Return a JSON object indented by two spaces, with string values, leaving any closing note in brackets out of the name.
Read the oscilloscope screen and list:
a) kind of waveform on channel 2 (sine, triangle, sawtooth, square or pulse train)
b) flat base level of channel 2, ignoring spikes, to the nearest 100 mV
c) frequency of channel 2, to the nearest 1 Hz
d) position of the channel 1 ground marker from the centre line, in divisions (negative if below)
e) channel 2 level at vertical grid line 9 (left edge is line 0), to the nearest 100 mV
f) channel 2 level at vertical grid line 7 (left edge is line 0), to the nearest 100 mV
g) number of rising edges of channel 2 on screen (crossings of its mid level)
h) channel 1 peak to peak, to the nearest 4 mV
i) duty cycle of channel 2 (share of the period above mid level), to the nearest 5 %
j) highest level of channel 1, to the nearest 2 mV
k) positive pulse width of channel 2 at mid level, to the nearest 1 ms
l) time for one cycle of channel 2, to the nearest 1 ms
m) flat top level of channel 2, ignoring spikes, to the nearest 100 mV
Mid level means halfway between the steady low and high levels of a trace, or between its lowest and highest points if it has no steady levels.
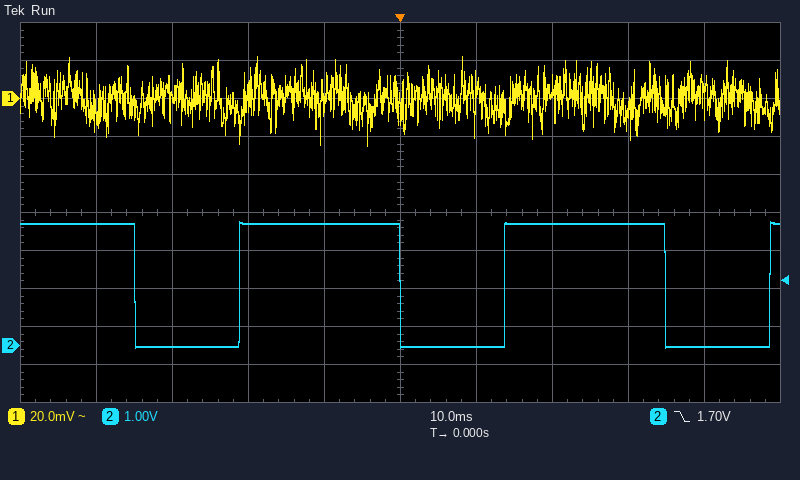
{
  "kind of waveform on channel 2": "pulse train",
  "flat base level of channel 2, ignoring spikes, to the nearest 100 mV": "0.0 V",
  "frequency of channel 2, to the nearest 1 Hz": "29 Hz",
  "position of the channel 1 ground marker from the centre line, in divisions": "+3.0 div",
  "channel 2 level at vertical grid line 9 (left edge is line 0), to the nearest 100 mV": "0.0 V",
  "channel 2 level at vertical grid line 7 (left edge is line 0), to the nearest 100 mV": "3.2 V",
  "number of rising edges of channel 2 on screen": "3",
  "channel 1 peak to peak, to the nearest 4 mV": "48 mV",
  "duty cycle of channel 2 (share of the period above mid level), to the nearest 5 %": "60 %",
  "highest level of channel 1, to the nearest 2 mV": "22 mV",
  "positive pulse width of channel 2 at mid level, to the nearest 1 ms": "21 ms",
  "time for one cycle of channel 2, to the nearest 1 ms": "35 ms",
  "flat top level of channel 2, ignoring spikes, to the nearest 100 mV": "3.2 V"
}
